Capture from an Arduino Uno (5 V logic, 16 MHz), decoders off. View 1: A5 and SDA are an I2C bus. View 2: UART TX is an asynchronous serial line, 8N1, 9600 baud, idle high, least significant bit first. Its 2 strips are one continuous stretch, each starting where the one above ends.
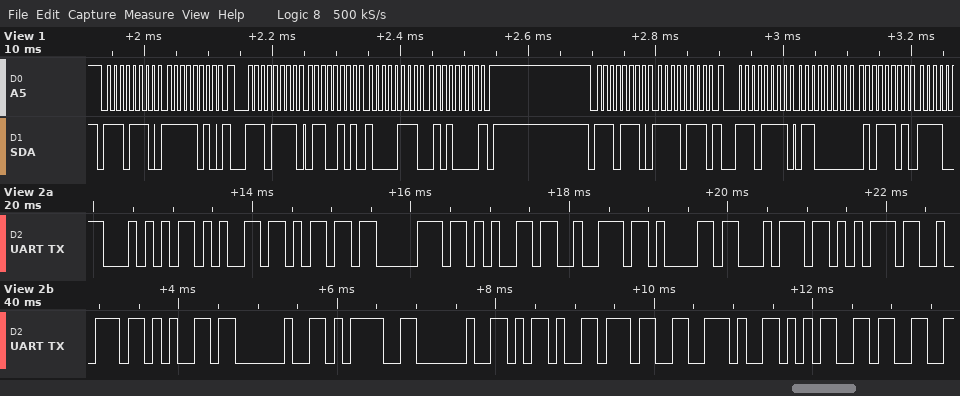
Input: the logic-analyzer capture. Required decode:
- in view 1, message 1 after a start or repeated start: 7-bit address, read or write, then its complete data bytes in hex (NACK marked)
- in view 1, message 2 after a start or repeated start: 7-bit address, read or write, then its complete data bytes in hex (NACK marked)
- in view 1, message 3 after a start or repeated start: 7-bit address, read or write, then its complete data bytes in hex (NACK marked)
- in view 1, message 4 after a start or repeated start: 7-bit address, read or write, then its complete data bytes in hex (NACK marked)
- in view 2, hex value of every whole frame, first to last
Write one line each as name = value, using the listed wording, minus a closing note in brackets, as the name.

in view 1, message 1 after a start or repeated start: 7-bit address, read or write, then its complete data bytes in hex = 0x77 write: FA
in view 1, message 2 after a start or repeated start: 7-bit address, read or write, then its complete data bytes in hex = 0x77 read: 65 87 50 NACK
in view 1, message 3 after a start or repeated start: 7-bit address, read or write, then its complete data bytes in hex = 0x77 write: F7
in view 1, message 4 after a start or repeated start: 7-bit address, read or write, then its complete data bytes in hex = 0x77 read: 60 5D
in view 2, hex value of every whole frame, first to last = 54 65 6D 70 65 72 61 74 75 72 65 20 3D 20 2D 37 2E 35 33
